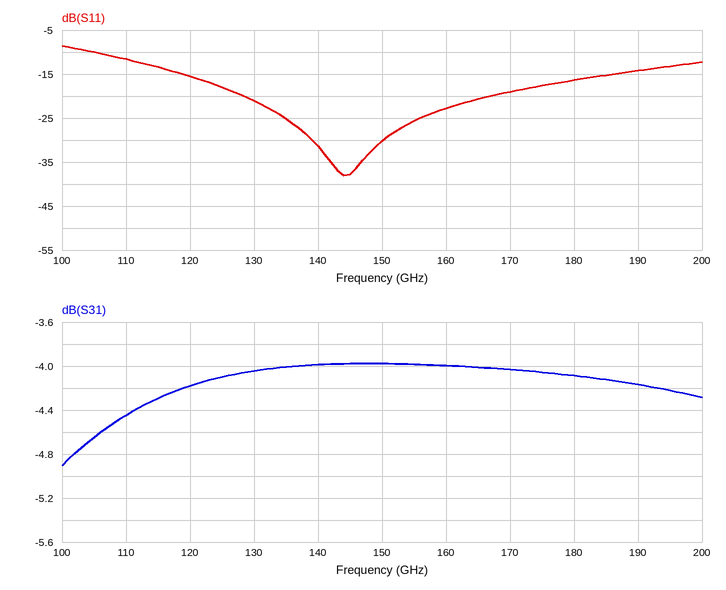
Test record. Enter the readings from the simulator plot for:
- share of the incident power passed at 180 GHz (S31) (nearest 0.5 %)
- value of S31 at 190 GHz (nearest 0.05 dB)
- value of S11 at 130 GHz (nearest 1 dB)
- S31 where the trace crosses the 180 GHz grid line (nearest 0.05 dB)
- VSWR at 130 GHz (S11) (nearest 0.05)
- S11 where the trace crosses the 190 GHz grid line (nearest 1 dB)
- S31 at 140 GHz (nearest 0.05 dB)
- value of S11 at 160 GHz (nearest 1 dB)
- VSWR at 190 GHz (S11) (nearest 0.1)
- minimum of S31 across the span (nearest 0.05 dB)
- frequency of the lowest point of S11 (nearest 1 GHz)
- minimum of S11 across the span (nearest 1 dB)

39.0 %
-4.15 dB
-21 dB
-4.10 dB
1.20
-14 dB
-4.00 dB
-23 dB
1.5
-4.90 dB
144 GHz
-38 dB
